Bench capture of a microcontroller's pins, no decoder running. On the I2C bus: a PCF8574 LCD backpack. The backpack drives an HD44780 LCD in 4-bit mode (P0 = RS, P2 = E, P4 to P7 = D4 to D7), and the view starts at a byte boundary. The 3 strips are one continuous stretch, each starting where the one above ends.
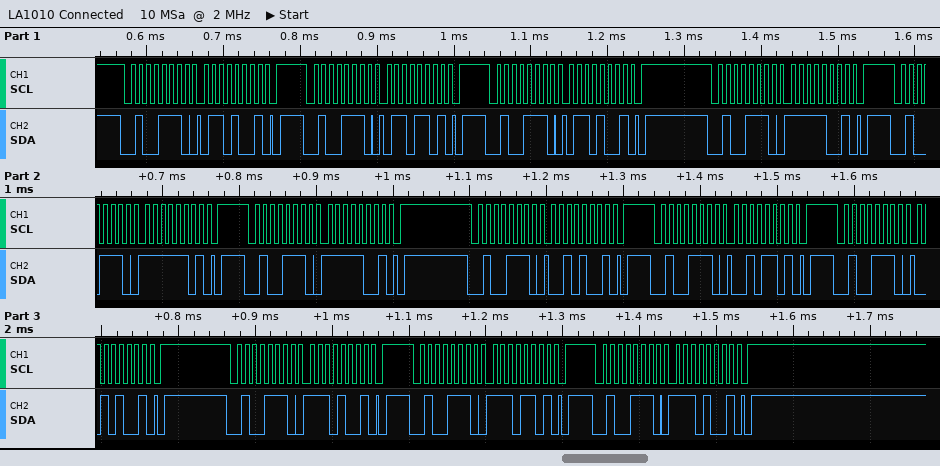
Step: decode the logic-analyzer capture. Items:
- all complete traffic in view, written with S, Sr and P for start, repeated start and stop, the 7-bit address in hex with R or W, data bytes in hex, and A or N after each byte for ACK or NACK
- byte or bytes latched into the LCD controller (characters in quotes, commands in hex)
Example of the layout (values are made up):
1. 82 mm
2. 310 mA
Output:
1. S 27W A 69 A P S 27W A 6D A P S 27W A 69 A P S 27W A F9 A P S 27W A FD A P S 27W A F9 A P S 27W A 29 A P S 27W A 2D A P S 27W A 29 A P S 27W A E9 A P S 27W A ED A P S 27W A E9 A P
2. 'o' '.'
